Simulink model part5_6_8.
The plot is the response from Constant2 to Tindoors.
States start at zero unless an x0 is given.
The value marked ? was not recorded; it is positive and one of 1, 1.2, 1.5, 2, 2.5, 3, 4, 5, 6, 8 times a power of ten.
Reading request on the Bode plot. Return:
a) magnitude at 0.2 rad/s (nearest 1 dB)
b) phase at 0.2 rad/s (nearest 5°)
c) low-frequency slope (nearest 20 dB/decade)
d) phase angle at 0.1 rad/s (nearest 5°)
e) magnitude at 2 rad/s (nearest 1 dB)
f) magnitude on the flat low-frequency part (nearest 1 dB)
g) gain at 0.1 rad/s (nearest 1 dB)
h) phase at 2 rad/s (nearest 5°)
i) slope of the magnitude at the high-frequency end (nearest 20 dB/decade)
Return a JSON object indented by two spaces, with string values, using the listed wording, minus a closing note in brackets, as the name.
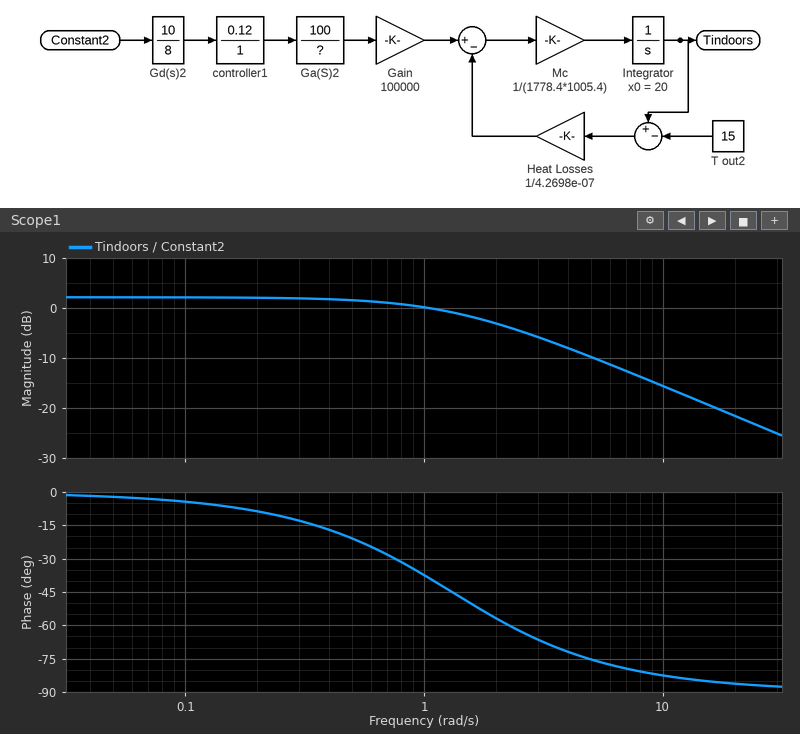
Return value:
{
  "magnitude at 0.2 rad/s": "2 dB",
  "phase at 0.2 rad/s": "-10°",
  "low-frequency slope": "0 dB/decade",
  "phase angle at 0.1 rad/s": "-5°",
  "magnitude at 2 rad/s": "-3 dB",
  "magnitude on the flat low-frequency part": "2 dB",
  "gain at 0.1 rad/s": "2 dB",
  "phase at 2 rad/s": "-55°",
  "slope of the magnitude at the high-frequency end": "-20 dB/decade"
}
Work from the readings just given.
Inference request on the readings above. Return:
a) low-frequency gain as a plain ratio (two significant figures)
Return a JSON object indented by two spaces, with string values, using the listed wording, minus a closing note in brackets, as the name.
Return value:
{
  "low-frequency gain as a plain ratio": "1.3"
}
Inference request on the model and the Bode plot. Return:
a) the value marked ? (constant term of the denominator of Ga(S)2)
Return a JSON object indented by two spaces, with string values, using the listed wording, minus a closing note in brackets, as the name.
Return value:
{
  "the value marked ? (constant term of the denominator of Ga(S)2)": "0.5"
}
